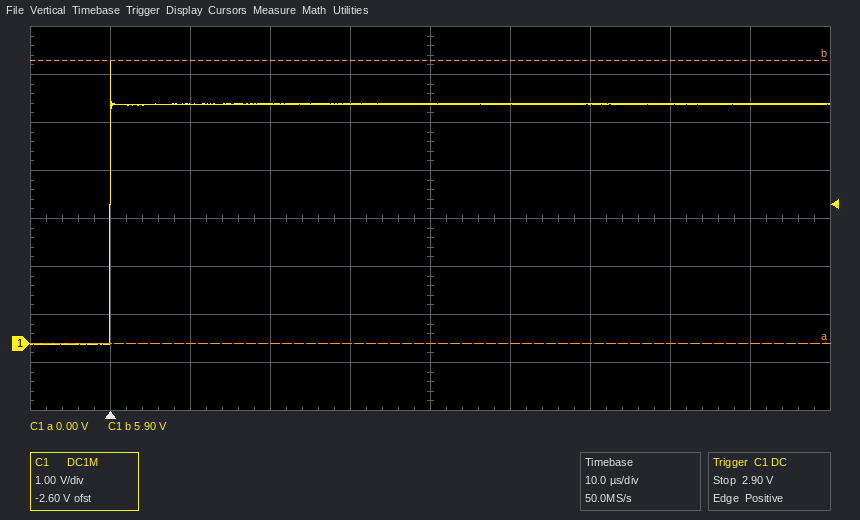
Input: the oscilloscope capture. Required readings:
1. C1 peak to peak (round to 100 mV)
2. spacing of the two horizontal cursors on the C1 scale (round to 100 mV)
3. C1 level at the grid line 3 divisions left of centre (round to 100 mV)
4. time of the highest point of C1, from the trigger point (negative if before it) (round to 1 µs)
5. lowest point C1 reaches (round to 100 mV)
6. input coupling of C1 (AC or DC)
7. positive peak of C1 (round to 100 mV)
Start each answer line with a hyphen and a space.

- 5.9 V
- 5.9 V
- 5.0 V
- 0 µs
- 0.0 V
- DC
- 5.9 V
